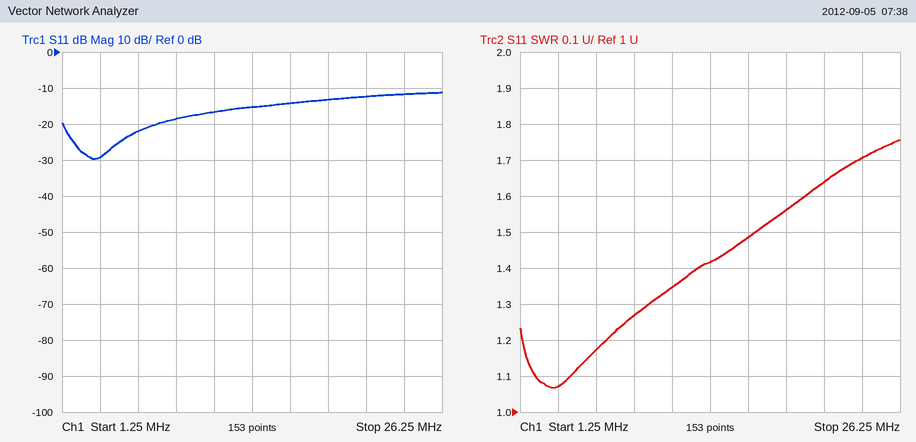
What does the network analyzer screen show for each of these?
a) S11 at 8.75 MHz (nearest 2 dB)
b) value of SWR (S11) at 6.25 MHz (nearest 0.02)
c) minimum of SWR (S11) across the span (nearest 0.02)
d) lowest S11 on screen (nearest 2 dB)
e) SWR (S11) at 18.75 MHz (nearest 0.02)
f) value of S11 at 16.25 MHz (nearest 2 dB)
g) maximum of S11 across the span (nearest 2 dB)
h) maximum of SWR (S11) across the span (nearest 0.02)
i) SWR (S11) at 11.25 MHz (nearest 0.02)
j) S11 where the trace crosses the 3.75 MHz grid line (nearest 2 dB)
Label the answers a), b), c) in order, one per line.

a) -18 dB
b) 1.18
c) 1.06
d) -30 dB
e) 1.56
f) -14 dB
g) -12 dB
h) 1.76
i) 1.34
j) -30 dB
